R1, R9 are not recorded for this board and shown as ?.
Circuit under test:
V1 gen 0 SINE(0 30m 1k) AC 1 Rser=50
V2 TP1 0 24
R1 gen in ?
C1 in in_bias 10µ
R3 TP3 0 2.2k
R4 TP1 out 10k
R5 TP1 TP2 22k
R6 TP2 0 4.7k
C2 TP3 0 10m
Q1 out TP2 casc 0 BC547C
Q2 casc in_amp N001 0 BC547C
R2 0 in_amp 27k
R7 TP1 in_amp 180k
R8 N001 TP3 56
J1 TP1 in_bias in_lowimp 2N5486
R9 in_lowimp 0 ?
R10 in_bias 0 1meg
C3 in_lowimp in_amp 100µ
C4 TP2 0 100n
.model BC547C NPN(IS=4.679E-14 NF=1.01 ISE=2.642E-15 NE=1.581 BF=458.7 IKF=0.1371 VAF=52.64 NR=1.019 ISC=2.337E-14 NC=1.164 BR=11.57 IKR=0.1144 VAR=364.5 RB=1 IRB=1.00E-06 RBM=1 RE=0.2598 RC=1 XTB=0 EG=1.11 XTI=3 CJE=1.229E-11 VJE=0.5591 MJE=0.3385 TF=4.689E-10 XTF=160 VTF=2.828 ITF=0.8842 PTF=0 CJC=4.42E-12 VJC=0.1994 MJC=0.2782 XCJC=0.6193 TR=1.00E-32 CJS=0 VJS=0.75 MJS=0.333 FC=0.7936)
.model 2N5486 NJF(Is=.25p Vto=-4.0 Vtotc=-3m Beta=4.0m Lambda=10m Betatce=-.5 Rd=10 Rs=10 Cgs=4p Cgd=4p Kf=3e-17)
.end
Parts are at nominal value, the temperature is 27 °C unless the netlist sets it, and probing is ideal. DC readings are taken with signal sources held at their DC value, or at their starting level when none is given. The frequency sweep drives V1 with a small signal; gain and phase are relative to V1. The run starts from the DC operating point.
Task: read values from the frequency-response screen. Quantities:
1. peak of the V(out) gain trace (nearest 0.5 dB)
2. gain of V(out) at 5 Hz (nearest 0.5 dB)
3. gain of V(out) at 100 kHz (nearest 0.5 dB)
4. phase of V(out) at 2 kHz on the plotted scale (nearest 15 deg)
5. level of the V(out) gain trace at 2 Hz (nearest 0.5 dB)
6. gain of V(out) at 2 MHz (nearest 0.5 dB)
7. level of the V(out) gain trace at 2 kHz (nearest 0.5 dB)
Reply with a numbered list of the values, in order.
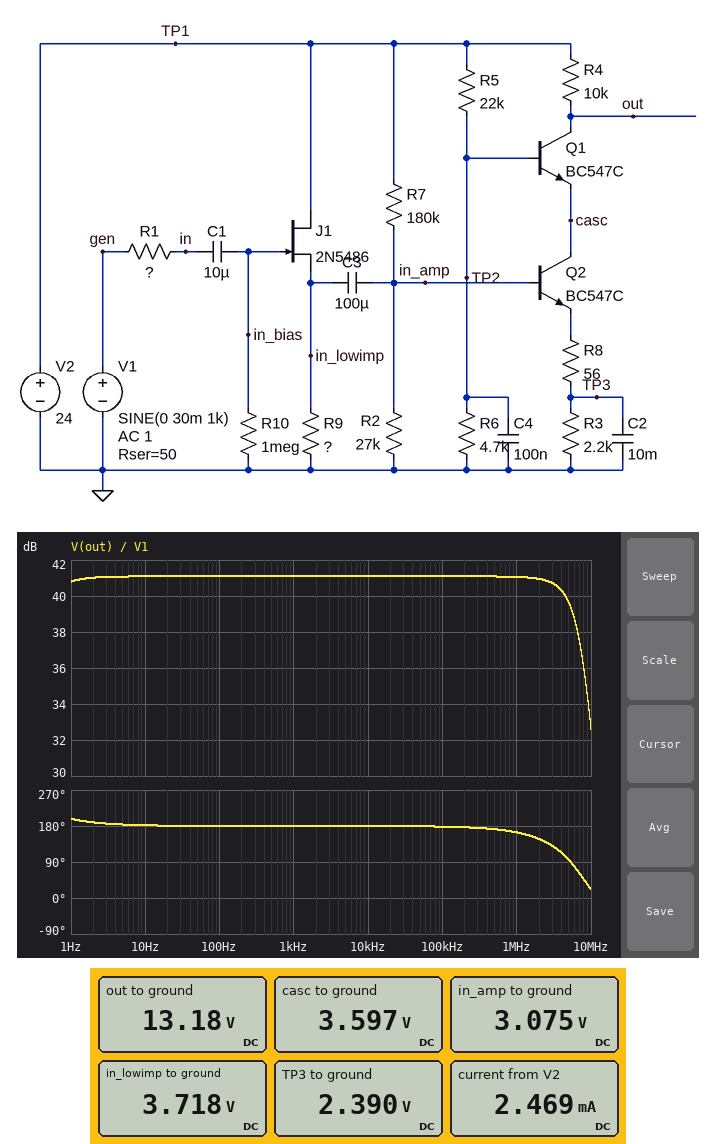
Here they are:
1. 41.0 dB
2. 41.0 dB
3. 41.0 dB
4. 180 deg
5. 41.0 dB
6. 41.0 dB
7. 41.0 dB
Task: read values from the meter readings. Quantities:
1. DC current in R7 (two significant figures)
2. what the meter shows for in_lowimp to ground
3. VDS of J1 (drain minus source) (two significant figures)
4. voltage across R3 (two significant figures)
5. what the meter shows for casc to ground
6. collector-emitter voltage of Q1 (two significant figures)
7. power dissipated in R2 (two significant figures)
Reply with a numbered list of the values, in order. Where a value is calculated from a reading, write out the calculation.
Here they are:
1. (24 V - 3.075 V) / 180 kΩ = 120 µA
2. 3.718 V
3. 24 V - 3.718 V = 20 V
4. 2.39 V = 2.4 V
5. 3.597 V
6. 13.18 V - 3.597 V = 9.6 V
7. (3.075 V)^2 / 27 kΩ = 350 µW
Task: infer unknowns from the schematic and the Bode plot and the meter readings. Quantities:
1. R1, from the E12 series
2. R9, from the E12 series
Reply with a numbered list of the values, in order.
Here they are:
1. 22 kΩ
2. 10 kΩ
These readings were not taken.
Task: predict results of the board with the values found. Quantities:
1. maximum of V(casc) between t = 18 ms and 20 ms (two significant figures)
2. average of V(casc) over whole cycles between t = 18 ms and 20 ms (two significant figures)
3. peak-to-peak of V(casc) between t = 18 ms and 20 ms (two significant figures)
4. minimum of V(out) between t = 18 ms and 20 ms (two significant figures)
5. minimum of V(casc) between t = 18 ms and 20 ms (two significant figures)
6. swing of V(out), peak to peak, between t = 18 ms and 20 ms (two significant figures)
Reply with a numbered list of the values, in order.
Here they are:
1. 3.6 V
2. 3.6 V
3. 21 mV
4. 9.6 V
5. 3.6 V
6. 6.8 V
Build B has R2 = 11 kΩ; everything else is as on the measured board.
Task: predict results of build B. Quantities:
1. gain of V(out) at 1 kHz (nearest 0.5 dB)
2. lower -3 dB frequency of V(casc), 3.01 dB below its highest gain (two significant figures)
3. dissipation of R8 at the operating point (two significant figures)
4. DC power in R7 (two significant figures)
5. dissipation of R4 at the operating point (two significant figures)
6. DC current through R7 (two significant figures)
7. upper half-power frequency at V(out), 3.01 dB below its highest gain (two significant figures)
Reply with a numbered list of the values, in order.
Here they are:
1. 36.5 dB
2. 240 mHz
3. 6.7 µW
4. 2.8 mW
5. 1.2 mW
6. 130 µA
7. 6.4 MHz
